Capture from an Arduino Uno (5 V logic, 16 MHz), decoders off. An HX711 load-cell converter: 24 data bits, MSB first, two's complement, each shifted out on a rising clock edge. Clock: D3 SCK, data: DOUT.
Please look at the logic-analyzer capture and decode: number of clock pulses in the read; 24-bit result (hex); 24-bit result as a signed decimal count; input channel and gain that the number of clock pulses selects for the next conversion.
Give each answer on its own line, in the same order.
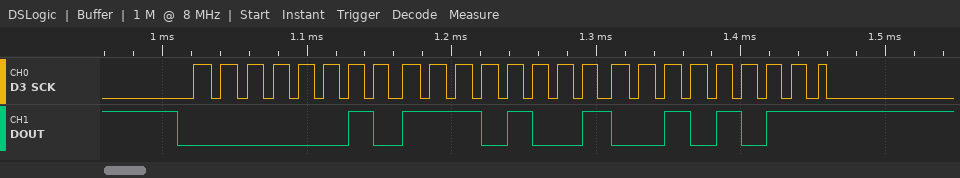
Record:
25
0x02E92B
190763
channel A, gain 128
